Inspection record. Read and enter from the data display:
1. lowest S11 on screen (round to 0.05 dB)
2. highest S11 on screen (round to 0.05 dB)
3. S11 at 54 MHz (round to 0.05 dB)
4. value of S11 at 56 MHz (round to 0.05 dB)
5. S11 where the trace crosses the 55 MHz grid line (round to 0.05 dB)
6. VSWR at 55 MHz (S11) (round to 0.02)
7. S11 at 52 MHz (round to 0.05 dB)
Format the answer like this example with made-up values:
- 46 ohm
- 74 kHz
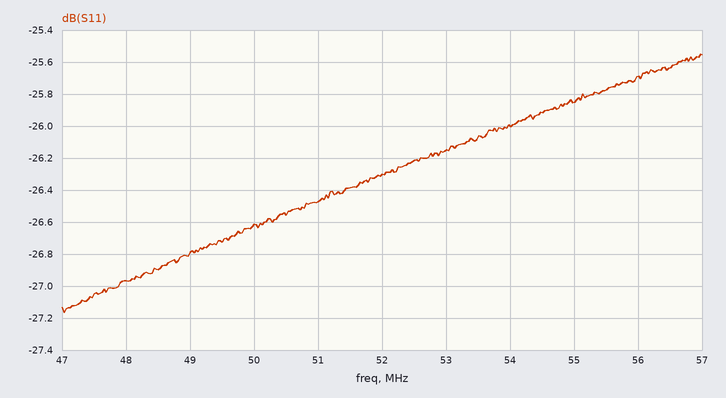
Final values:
- -27.15 dB
- -25.55 dB
- -26.00 dB
- -25.70 dB
- -25.85 dB
- 1.10
- -26.30 dB
